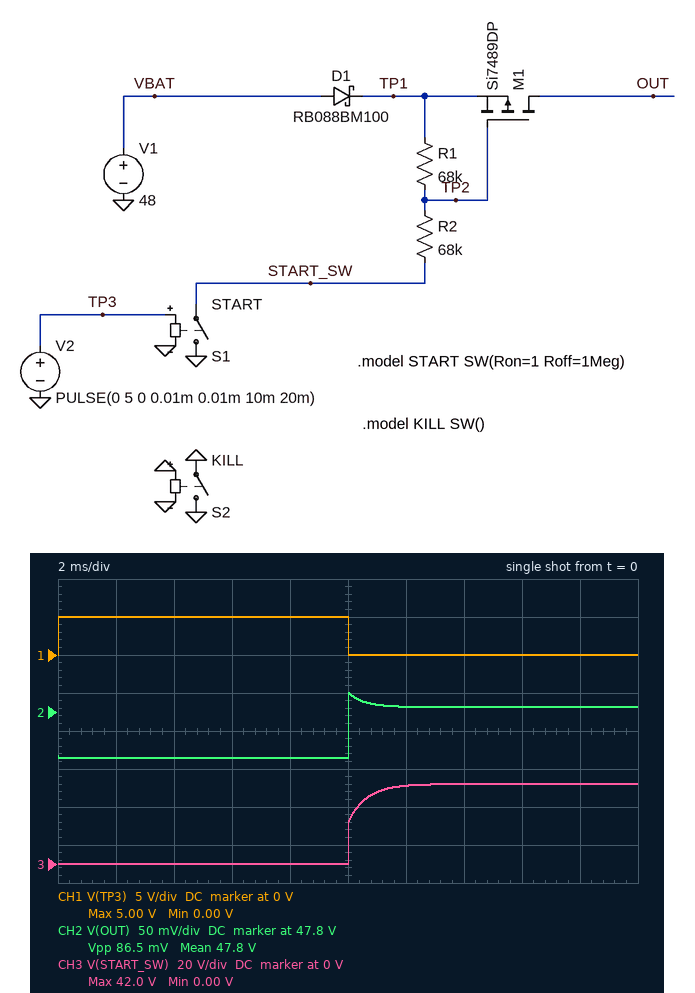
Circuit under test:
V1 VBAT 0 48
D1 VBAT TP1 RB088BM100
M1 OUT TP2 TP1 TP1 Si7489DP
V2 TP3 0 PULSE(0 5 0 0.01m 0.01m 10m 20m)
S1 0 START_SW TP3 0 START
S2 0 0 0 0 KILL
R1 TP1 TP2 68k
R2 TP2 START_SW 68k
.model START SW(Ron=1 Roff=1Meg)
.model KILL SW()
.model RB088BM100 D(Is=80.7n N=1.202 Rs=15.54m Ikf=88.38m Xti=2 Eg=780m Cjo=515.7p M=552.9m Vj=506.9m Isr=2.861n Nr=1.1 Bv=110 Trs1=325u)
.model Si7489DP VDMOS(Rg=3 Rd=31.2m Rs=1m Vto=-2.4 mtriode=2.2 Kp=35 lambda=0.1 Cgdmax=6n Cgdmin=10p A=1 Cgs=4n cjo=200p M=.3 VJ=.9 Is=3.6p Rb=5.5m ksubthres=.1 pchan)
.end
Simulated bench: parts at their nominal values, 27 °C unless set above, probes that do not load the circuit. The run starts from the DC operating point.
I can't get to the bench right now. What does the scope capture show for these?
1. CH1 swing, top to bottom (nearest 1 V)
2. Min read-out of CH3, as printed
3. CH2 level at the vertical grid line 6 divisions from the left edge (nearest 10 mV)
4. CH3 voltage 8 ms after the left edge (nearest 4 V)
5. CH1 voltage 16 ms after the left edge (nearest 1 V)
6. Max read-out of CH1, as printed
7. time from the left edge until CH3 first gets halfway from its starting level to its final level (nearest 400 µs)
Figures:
5 V
0.00 V
47.81 V
0 V
0 V
5.00 V
10.0 ms
